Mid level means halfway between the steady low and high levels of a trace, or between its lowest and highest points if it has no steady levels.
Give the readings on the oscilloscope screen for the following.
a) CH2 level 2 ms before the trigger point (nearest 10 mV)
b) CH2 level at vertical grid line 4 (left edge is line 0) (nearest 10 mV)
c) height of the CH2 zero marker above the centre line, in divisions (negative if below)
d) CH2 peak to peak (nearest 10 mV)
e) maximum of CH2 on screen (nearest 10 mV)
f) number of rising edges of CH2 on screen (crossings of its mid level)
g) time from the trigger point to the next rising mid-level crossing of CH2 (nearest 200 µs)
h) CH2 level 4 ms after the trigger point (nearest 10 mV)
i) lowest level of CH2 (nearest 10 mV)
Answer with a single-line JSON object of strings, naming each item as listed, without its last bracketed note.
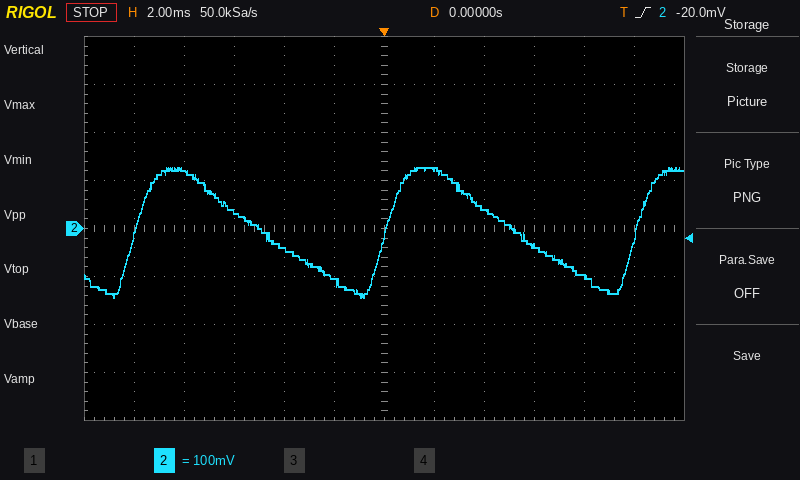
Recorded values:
{"CH2 level 2 ms before the trigger point": "-110 mV", "CH2 level at vertical grid line 4 (left edge is line 0)": "-40 mV", "height of the CH2 zero marker above the centre line, in divisions": "0.0 div", "CH2 peak to peak": "270 mV", "maximum of CH2 on screen": "130 mV", "number of rising edges of CH2 on screen": "3", "time from the trigger point to the next rising mid-level crossing of CH2": "10.0 ms", "CH2 level 4 ms after the trigger point": "40 mV", "lowest level of CH2": "-140 mV"}
